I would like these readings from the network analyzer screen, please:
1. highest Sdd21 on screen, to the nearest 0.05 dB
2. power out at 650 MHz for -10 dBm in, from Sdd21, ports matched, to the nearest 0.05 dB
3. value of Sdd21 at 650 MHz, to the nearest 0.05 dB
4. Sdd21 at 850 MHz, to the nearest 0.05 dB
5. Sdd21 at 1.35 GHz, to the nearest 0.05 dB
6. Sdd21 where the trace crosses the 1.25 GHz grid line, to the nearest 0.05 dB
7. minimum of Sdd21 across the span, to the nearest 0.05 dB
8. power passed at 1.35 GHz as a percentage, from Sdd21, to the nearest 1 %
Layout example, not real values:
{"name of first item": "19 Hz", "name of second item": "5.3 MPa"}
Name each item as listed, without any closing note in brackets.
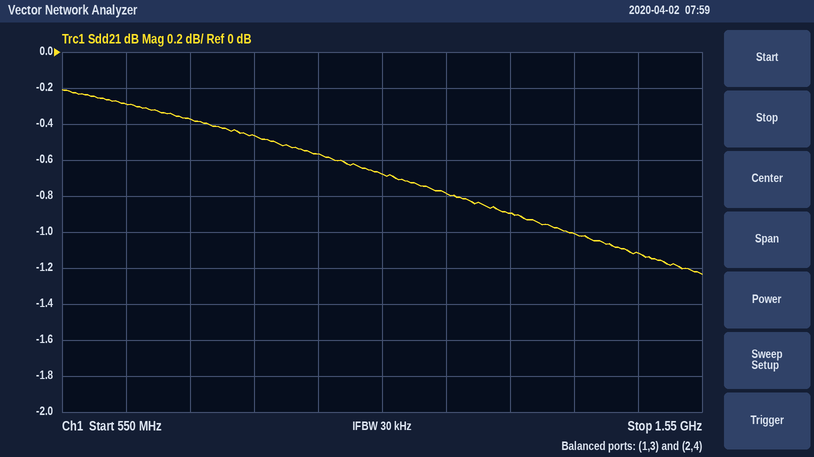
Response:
{"highest Sdd21 on screen, to the nearest 0.05 dB": "-0.20 dB", "power out at 650 MHz for -10 dBm in, from Sdd21, ports matched, to the nearest 0.05 dB": "-10.30 dBm", "value of Sdd21 at 650 MHz, to the nearest 0.05 dB": "-0.30 dB", "Sdd21 at 850 MHz, to the nearest 0.05 dB": "-0.45 dB", "Sdd21 at 1.35 GHz, to the nearest 0.05 dB": "-1.00 dB", "Sdd21 where the trace crosses the 1.25 GHz grid line, to the nearest 0.05 dB": "-0.90 dB", "minimum of Sdd21 across the span, to the nearest 0.05 dB": "-1.25 dB", "power passed at 1.35 GHz as a percentage, from Sdd21, to the nearest 1 %": "79 %"}
